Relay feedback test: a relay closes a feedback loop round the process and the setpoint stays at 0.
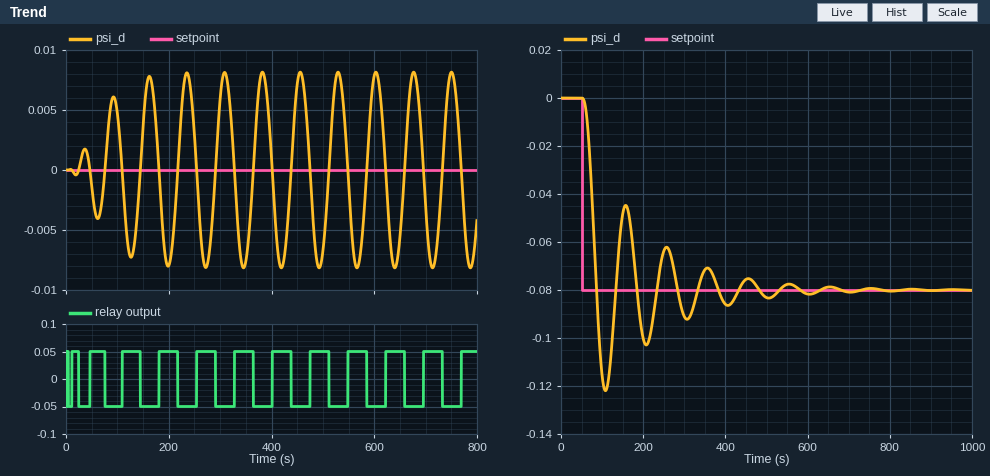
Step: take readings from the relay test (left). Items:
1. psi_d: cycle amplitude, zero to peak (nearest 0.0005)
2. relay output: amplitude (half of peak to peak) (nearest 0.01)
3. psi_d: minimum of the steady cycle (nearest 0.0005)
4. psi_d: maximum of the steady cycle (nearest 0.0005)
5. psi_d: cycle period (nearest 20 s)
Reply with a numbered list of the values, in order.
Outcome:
1. 0.0080
2. 0.05
3. -0.0080
4. 0.0080
5. 80 s
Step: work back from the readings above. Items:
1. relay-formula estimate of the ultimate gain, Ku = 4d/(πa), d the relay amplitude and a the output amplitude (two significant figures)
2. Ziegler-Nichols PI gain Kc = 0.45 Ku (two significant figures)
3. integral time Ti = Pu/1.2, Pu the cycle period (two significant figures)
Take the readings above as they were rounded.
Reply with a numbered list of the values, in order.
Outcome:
1. 8.0
2. 3.6
3. 67 s
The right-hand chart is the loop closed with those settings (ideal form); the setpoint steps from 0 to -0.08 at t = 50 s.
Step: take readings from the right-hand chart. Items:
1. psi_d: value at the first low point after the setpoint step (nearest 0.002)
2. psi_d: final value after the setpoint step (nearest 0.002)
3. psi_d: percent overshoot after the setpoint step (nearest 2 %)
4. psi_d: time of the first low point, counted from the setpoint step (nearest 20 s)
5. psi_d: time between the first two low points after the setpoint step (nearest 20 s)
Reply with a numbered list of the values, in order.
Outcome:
1. -0.122
2. -0.080
3. 52 %
4. 60 s
5. 100 s
